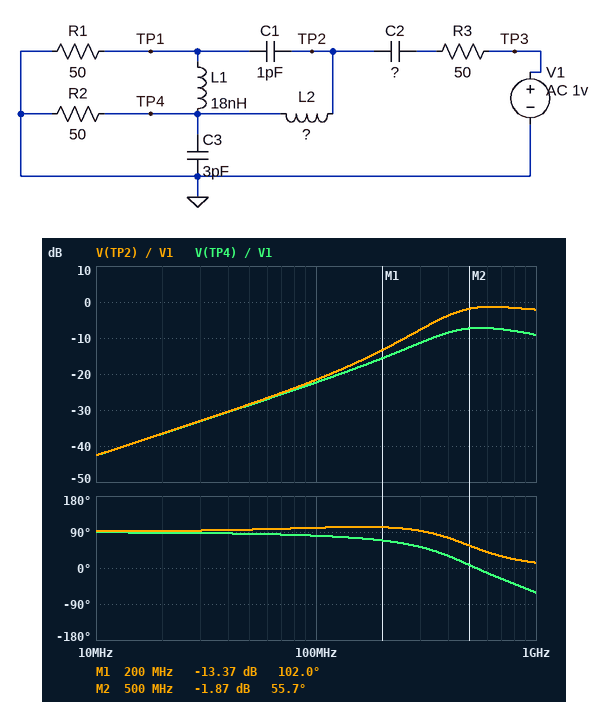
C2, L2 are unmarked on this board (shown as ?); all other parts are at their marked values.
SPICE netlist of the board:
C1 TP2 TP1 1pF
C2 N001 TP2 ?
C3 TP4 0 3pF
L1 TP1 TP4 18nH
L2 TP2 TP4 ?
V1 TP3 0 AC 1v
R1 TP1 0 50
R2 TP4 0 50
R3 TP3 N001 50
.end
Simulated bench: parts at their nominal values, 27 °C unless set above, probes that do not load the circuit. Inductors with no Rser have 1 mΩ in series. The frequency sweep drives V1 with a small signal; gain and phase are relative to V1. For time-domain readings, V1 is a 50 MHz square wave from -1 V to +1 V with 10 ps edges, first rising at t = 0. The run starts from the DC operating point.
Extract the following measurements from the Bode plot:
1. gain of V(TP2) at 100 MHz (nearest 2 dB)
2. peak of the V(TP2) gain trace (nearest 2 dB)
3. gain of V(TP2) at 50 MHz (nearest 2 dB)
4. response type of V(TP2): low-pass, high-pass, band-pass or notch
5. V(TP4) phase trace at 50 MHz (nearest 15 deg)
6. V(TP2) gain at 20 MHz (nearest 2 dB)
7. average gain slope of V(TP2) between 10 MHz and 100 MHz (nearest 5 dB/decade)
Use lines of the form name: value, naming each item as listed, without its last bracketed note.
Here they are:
gain of V(TP2) at 100 MHz: -22 dB
peak of the V(TP2) gain trace: -2 dB
gain of V(TP2) at 50 MHz: -28 dB
response type of V(TP2): low-pass, high-pass, band-pass or notch: high-pass
V(TP4) phase trace at 50 MHz: 90 deg
V(TP2) gain at 20 MHz: -36 dB
average gain slope of V(TP2) between 10 MHz and 100 MHz: 20 dB/decade
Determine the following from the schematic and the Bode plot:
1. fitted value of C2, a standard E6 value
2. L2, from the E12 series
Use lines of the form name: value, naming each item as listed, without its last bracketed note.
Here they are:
fitted value of C2, a standard E6 value: 4.7 pF
L2, from the E12 series: 15 nH
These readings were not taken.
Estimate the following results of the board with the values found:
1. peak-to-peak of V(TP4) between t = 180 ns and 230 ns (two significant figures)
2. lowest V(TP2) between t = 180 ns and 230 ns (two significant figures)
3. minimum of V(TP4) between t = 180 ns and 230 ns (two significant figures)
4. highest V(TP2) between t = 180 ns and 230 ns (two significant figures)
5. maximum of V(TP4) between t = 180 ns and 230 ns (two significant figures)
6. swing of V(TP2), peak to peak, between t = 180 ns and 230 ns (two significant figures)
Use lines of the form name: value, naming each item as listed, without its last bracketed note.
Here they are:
peak-to-peak of V(TP4) between t = 180 ns and 230 ns: 1.1 V
lowest V(TP2) between t = 180 ns and 230 ns: -1.2 V
minimum of V(TP4) between t = 180 ns and 230 ns: -530 mV
highest V(TP2) between t = 180 ns and 230 ns: 1.2 V
maximum of V(TP4) between t = 180 ns and 230 ns: 530 mV
swing of V(TP2), peak to peak, between t = 180 ns and 230 ns: 2.3 V
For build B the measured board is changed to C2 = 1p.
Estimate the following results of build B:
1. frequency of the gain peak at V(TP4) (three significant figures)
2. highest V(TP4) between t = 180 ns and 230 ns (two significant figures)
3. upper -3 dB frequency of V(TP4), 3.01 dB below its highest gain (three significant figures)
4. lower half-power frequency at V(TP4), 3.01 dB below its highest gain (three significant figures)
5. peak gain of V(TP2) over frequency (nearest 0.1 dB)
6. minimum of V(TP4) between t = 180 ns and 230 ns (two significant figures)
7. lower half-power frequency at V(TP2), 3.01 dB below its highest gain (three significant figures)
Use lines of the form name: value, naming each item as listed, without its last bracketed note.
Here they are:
frequency of the gain peak at V(TP4): 827 MHz
highest V(TP4) between t = 180 ns and 230 ns: 270 mV
upper -3 dB frequency of V(TP4), 3.01 dB below its highest gain: 1.29 GHz
lower half-power frequency at V(TP4), 3.01 dB below its highest gain: 607 MHz
peak gain of V(TP2) over frequency: -3.1 dB
minimum of V(TP4) between t = 180 ns and 230 ns: -270 mV
lower half-power frequency at V(TP2), 3.01 dB below its highest gain: 626 MHz
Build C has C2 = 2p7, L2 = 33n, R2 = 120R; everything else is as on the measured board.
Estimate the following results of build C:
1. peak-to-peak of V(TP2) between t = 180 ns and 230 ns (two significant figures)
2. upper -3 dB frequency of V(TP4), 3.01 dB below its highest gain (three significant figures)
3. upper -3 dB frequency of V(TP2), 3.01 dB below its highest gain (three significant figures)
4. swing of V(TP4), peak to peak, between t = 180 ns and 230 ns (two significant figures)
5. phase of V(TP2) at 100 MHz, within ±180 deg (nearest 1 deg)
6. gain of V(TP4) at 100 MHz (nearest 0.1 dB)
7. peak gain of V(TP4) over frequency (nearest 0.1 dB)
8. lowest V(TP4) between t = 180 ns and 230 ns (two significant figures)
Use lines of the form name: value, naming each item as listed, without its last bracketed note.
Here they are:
peak-to-peak of V(TP2) between t = 180 ns and 230 ns: 2.3 V
upper -3 dB frequency of V(TP4), 3.01 dB below its highest gain: 647 MHz
upper -3 dB frequency of V(TP2), 3.01 dB below its highest gain: 671 MHz
swing of V(TP4), peak to peak, between t = 180 ns and 230 ns: 980 mV
phase of V(TP2) at 100 MHz, within ±180 deg: 115 deg
gain of V(TP4) at 100 MHz: -23.9 dB
peak gain of V(TP4) over frequency: -5.4 dB
lowest V(TP4) between t = 180 ns and 230 ns: -490 mV
